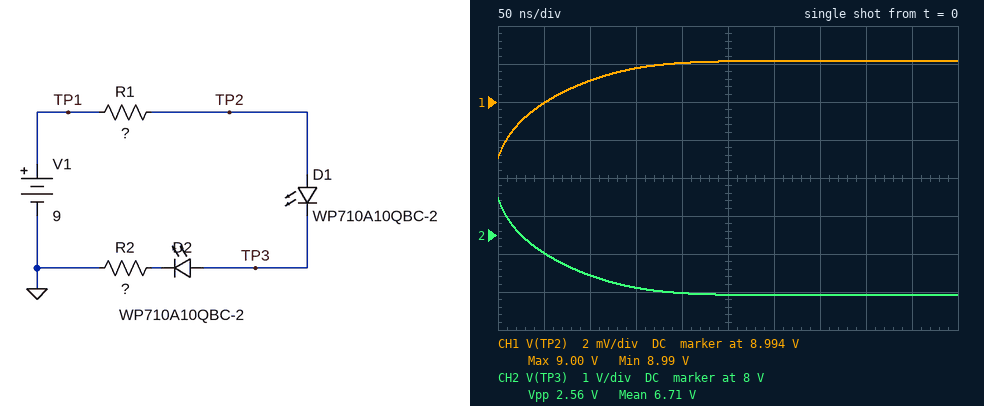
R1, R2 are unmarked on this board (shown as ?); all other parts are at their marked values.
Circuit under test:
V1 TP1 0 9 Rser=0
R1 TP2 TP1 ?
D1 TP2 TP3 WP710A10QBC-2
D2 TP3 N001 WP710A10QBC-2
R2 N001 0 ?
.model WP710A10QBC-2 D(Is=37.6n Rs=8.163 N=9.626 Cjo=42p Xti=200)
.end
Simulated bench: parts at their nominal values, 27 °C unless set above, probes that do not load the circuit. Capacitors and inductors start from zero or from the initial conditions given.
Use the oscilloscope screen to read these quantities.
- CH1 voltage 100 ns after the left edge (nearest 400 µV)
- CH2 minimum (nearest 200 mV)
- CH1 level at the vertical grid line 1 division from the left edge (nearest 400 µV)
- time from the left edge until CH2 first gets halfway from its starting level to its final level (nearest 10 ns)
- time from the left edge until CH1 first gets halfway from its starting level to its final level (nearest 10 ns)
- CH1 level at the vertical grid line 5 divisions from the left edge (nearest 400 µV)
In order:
8.9952 V
6.4 V
8.9940 V
40 ns
40 ns
8.9960 V
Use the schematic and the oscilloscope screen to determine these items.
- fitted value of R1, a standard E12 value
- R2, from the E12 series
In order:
3.3 Ω
3.3 kΩ
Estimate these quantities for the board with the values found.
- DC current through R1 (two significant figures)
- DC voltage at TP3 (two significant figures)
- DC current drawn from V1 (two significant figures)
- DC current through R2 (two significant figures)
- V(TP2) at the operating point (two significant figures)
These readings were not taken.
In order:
1.2 mA
6.4 V
1.2 mA
1.2 mA
9.0 V
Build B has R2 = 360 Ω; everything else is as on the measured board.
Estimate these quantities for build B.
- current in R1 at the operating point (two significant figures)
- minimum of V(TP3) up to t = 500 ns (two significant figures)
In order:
7.7 mA
5.9 V
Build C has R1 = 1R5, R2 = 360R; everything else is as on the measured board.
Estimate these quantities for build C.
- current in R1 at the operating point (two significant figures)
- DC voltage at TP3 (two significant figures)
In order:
7.7 mA
5.9 V
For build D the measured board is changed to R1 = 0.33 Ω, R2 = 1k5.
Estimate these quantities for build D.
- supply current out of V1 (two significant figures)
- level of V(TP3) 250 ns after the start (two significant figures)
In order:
2.3 mA
6.2 V
